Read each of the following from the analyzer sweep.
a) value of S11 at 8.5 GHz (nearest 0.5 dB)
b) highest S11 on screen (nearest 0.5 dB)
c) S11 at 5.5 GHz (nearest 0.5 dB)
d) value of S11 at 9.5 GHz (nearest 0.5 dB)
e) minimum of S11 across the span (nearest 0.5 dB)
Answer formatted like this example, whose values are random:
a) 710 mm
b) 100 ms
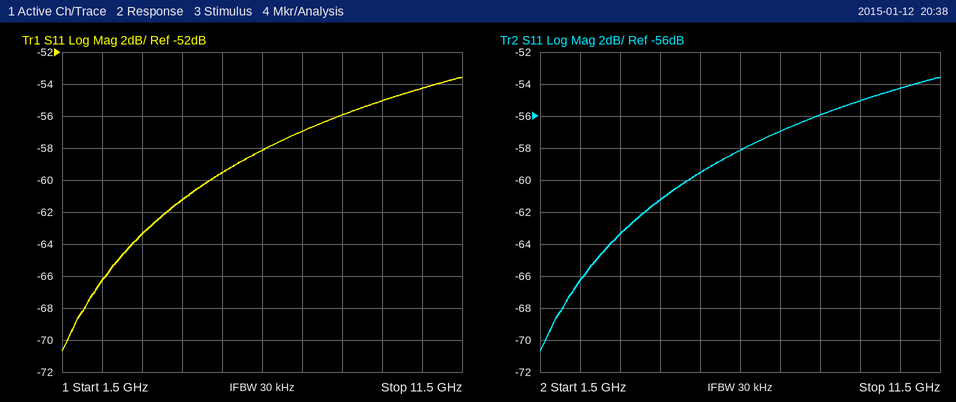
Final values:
a) -56.0 dB
b) -53.5 dB
c) -59.5 dB
d) -55.0 dB
e) -70.5 dB
